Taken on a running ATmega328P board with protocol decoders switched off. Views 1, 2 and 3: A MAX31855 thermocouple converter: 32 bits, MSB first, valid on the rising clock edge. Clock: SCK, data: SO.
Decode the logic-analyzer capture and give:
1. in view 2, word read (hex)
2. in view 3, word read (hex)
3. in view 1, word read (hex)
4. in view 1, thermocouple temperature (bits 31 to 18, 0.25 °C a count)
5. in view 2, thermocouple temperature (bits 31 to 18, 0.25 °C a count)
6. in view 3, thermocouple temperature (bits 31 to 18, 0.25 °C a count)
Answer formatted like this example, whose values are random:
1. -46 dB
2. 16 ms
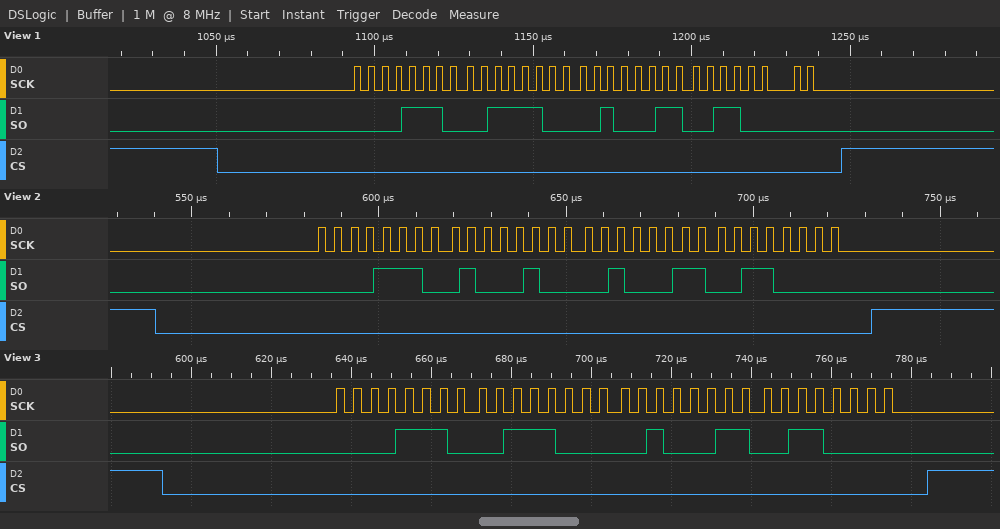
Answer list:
1. 0x0E442330
2. 0x0E382330
3. 0x0E3C2330
4. 227.75 °C
5. 228.25 °C
6. 227.50 °C
